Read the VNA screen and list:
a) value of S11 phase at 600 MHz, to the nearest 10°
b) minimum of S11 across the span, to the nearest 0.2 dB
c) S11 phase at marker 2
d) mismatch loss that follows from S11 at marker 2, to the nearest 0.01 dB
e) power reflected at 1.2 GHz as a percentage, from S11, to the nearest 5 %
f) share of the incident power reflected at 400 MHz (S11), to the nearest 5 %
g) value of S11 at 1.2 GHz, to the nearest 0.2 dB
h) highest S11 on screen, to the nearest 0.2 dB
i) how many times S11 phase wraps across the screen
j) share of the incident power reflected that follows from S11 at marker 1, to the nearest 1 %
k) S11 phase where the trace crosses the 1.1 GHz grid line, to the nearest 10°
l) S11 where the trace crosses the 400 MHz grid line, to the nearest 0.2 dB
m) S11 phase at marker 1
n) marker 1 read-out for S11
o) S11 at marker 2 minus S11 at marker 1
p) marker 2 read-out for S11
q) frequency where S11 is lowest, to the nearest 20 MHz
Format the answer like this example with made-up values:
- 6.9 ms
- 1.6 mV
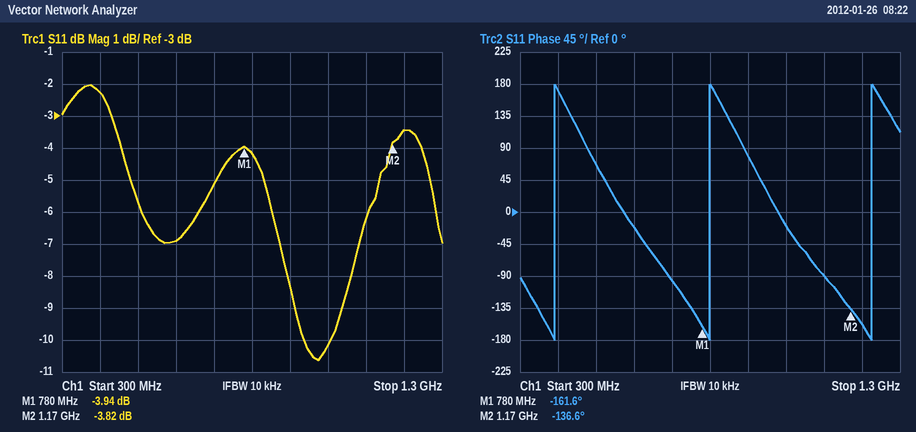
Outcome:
- -20°
- -10.6 dB
- -136.6°
- 2.33 dB
- 45 %
- 60 %
- -3.4 dB
- -2.0 dB
- 3
- 40 %
- -90°
- -2.2 dB
- -161.6°
- -3.94 dB
- 0.12 dB
- -3.82 dB
- 980 MHz
